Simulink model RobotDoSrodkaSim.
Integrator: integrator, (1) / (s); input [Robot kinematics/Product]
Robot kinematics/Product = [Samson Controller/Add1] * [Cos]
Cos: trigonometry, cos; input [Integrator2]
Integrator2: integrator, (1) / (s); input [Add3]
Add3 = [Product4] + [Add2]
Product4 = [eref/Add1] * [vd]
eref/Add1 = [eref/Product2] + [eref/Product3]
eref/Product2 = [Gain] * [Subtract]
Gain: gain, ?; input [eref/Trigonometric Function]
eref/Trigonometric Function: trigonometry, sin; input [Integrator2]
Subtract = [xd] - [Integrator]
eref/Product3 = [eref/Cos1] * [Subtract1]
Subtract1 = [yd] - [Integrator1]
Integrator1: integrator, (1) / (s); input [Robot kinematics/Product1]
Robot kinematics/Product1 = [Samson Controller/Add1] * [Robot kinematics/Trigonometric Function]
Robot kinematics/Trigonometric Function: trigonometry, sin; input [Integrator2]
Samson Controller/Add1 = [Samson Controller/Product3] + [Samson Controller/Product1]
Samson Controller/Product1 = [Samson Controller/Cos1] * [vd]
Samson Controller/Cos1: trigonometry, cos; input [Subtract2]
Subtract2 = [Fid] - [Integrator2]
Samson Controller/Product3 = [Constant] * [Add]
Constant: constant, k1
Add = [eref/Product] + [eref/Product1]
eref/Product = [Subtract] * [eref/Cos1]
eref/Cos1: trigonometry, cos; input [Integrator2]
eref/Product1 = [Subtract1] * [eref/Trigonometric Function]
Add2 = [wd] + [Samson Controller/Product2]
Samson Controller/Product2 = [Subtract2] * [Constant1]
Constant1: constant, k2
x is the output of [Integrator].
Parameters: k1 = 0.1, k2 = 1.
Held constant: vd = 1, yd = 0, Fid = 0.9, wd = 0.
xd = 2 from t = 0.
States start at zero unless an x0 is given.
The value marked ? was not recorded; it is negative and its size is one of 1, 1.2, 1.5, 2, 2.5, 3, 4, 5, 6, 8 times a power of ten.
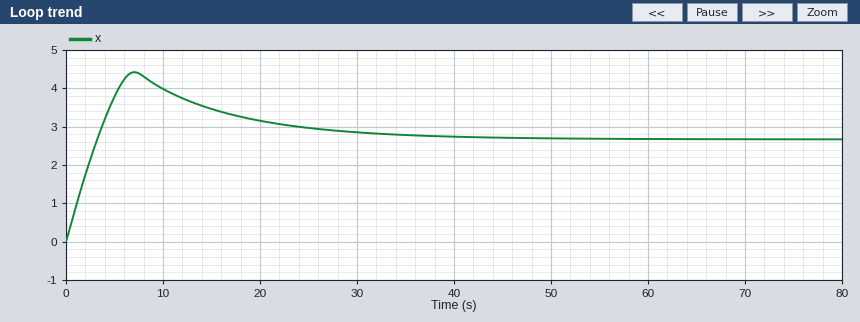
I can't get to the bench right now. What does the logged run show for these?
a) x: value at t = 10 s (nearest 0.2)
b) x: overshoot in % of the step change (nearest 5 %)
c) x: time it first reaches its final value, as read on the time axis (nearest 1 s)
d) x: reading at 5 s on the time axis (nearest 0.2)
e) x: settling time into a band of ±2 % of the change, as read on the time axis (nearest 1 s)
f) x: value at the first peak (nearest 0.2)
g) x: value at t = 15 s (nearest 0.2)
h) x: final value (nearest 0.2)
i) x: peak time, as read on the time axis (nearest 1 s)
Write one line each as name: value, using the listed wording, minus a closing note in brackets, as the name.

x: value at t = 10 s: 4.0
x: overshoot in % of the step change: 65 %
x: time it first reaches its final value, as read on the time axis: 3 s
x: reading at 5 s on the time axis: 3.8
x: settling time into a band of ±2 % of the change, as read on the time axis: 43 s
x: value at the first peak: 4.4
x: value at t = 15 s: 3.4
x: final value: 2.6
x: peak time, as read on the time axis: 7 s
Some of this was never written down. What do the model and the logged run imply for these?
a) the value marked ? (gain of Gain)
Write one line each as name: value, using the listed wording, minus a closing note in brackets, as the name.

the value marked ?: -0.8
